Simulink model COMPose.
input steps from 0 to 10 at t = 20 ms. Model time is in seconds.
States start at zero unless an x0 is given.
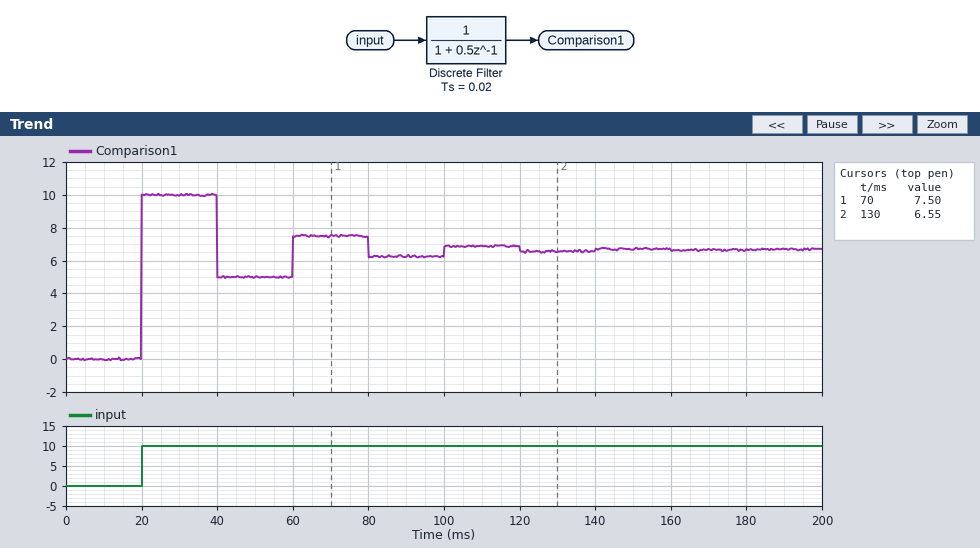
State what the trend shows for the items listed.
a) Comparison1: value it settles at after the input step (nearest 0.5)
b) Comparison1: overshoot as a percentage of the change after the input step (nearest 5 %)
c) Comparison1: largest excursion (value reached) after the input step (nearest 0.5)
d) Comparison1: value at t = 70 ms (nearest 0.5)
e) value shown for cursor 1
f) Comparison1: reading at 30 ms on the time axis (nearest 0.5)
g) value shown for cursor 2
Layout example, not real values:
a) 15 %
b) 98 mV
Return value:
a) 6.5
b) 50 %
c) 10.0
d) 7.5
e) 7.50
f) 10.0
g) 6.55
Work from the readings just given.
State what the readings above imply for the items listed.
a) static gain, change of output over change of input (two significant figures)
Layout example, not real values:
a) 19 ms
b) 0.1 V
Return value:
a) 0.65
